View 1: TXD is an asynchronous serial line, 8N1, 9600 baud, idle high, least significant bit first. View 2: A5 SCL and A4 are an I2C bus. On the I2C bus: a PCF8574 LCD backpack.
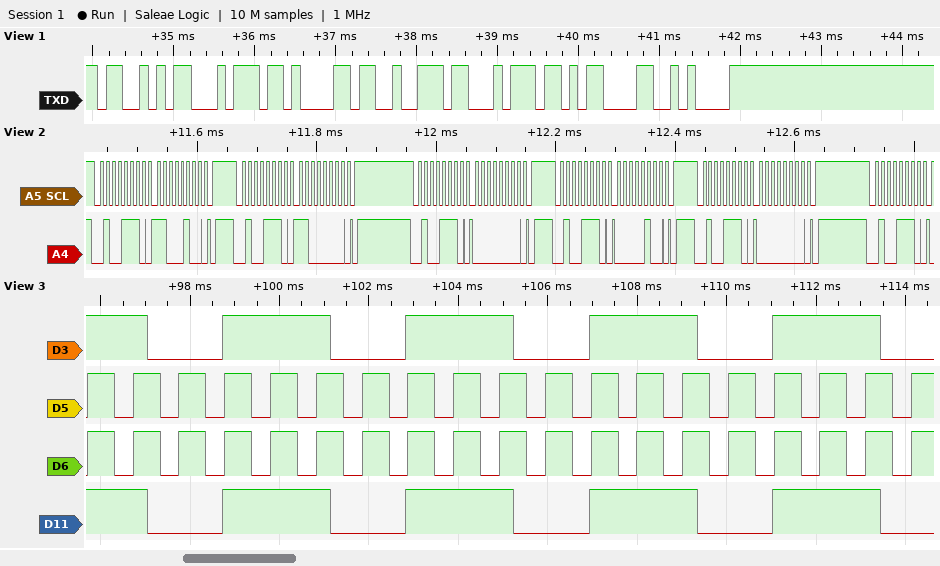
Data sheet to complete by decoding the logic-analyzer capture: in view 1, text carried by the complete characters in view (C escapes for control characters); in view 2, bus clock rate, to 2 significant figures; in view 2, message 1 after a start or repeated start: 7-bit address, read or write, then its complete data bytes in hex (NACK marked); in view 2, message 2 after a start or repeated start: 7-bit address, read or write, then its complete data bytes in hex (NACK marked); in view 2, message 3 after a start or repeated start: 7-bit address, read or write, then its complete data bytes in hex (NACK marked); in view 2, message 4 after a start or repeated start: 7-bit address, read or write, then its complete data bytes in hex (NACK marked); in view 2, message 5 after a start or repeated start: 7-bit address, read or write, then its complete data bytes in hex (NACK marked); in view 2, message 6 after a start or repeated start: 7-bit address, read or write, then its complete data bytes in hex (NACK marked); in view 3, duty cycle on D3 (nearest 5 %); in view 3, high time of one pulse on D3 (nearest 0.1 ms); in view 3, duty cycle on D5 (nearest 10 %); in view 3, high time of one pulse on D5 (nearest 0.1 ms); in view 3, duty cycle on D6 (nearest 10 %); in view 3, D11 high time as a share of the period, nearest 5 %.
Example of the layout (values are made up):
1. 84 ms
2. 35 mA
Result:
1. "Start\r\n"
2. 100 kHz
3. 0x27 write: C4
4. 0x27 write: C0
5. 0x27 write: 00
6. 0x27 write: 04
7. 0x27 write: 00
8. 0x27 write
9. 60 %
10. 2.4 ms
11. 60 %
12. 0.6 ms
13. 60 %
14. 60 %
